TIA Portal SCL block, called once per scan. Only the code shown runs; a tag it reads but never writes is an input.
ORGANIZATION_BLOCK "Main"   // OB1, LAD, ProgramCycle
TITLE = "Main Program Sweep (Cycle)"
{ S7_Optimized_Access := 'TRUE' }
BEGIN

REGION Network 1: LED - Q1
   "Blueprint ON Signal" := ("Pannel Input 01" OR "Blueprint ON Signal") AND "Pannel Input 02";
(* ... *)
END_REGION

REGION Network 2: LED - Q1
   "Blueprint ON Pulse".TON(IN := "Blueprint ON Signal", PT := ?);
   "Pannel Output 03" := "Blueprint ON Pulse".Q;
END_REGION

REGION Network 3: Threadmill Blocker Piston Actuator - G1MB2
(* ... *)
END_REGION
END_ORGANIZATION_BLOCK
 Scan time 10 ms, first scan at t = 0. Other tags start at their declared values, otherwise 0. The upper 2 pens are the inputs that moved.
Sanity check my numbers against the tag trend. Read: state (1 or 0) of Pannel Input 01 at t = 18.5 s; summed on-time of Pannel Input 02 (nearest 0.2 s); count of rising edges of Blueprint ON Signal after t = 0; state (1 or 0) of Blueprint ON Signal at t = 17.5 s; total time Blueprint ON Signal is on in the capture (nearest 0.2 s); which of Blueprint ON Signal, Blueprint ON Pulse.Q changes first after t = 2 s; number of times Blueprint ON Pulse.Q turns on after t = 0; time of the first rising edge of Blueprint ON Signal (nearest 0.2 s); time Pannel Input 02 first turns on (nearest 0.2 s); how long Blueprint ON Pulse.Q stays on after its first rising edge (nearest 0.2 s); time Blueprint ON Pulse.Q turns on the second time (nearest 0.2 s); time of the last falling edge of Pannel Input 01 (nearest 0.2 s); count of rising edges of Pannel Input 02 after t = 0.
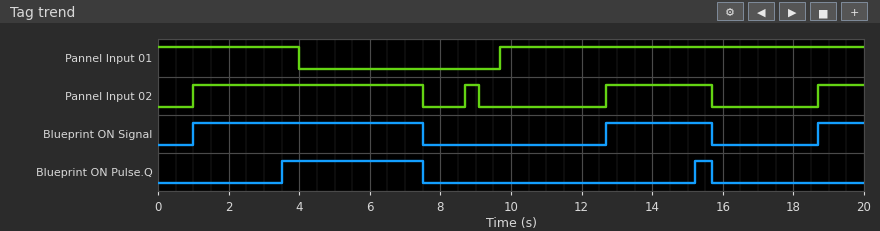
1
11.2 s
3
0
10.8 s
Blueprint ON Pulse.Q
2
1.0 s
1.0 s
4.0 s
15.2 s
4.0 s
4
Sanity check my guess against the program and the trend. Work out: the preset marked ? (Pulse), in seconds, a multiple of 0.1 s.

2.5 s
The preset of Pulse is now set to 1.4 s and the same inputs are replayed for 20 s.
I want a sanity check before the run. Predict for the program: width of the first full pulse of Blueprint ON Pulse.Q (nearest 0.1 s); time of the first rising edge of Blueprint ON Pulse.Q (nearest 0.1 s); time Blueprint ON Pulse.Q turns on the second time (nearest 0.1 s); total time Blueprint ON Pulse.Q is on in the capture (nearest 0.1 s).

5.1 s
2.4 s
14.1 s
6.7 s
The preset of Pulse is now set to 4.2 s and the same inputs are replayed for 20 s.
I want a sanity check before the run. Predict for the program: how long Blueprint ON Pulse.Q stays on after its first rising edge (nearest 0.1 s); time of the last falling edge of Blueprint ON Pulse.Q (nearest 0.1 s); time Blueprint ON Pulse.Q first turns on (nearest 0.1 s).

2.3 s
7.5 s
5.2 s
